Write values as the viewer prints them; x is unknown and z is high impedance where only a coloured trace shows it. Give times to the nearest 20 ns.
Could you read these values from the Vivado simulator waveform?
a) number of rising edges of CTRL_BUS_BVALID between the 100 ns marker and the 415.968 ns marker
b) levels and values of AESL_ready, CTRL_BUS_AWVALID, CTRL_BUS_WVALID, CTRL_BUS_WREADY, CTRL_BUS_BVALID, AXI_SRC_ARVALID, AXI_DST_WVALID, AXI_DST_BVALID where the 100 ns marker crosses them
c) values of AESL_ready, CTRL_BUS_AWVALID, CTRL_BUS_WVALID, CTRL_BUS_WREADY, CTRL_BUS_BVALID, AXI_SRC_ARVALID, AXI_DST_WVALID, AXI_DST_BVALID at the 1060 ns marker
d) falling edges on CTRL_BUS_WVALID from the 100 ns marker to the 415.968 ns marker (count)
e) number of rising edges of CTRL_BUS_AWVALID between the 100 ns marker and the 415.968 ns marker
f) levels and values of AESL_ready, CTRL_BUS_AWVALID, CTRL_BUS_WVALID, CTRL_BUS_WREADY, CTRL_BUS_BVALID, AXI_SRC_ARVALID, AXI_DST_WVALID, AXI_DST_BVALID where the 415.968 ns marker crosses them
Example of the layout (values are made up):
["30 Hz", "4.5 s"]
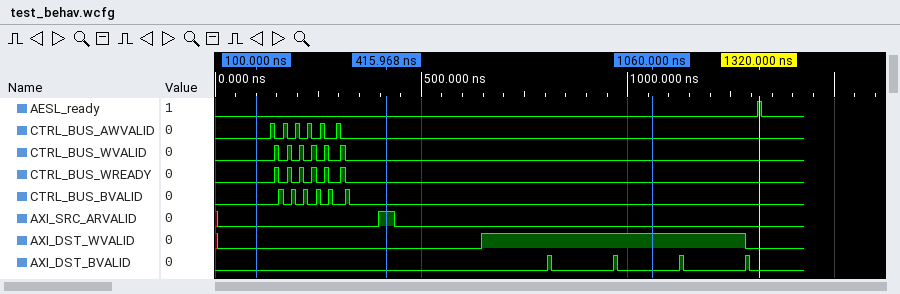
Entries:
["6", "AESL_ready=0, CTRL_BUS_AWVALID=0, CTRL_BUS_WVALID=0, CTRL_BUS_WREADY=0, CTRL_BUS_BVALID=0, AXI_SRC_ARVALID=0, AXI_DST_WVALID=0, AXI_DST_BVALID=0", "AESL_ready=0, CTRL_BUS_AWVALID=0, CTRL_BUS_WVALID=0, CTRL_BUS_WREADY=0, CTRL_BUS_BVALID=0, AXI_SRC_ARVALID=0, AXI_DST_WVALID=1, AXI_DST_BVALID=0", "6", "6", "AESL_ready=0, CTRL_BUS_AWVALID=0, CTRL_BUS_WVALID=0, CTRL_BUS_WREADY=0, CTRL_BUS_BVALID=0, AXI_SRC_ARVALID=1, AXI_DST_WVALID=0, AXI_DST_BVALID=0"]
